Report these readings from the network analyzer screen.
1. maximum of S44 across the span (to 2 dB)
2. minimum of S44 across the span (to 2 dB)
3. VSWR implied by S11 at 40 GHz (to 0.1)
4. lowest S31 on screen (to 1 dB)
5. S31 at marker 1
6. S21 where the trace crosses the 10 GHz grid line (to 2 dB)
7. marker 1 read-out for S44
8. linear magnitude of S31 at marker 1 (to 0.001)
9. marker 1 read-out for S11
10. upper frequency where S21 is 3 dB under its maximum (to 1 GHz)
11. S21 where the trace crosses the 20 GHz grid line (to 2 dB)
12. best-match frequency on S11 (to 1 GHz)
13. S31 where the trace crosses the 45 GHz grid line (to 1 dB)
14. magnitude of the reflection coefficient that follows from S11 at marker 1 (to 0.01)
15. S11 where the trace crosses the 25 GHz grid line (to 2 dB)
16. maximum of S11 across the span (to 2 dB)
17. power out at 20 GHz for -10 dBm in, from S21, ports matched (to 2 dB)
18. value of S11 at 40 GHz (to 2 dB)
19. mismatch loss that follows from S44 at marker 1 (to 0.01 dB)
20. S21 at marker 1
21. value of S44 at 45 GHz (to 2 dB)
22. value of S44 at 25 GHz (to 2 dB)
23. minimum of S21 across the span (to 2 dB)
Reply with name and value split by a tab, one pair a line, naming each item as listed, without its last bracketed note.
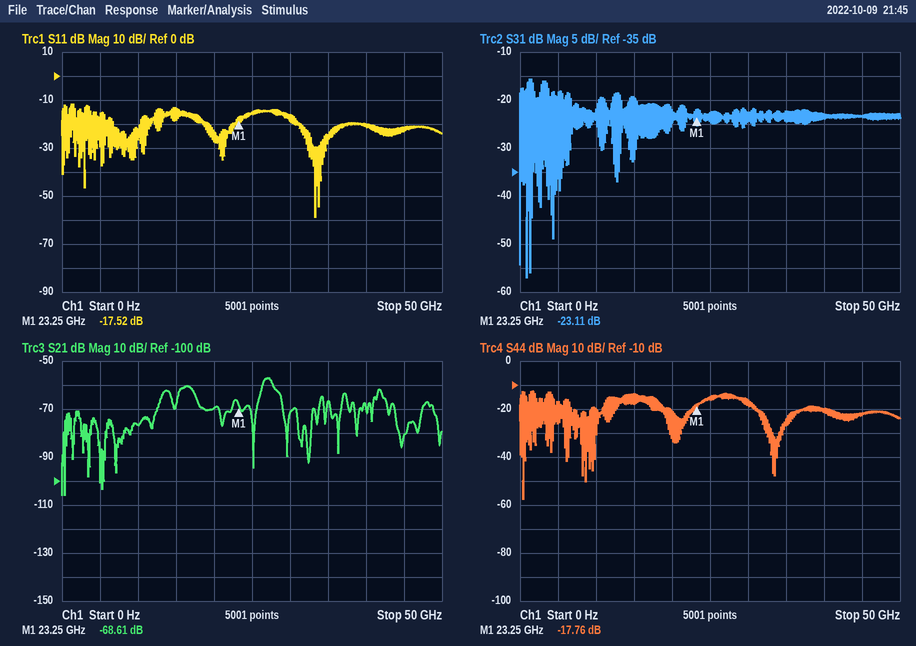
maximum of S44 across the span	-12 dB
minimum of S44 across the span	-58 dB
VSWR implied by S11 at 40 GHz	1.2
lowest S31 on screen	-57 dB
S31 at marker 1	-23.11 dB
S21 where the trace crosses the 10 GHz grid line	-76 dB
marker 1 read-out for S44	-17.76 dB
linear magnitude of S31 at marker 1	0.070
marker 1 read-out for S11	-17.52 dB
upper frequency where S21 is 3 dB under its maximum	28 GHz
S21 where the trace crosses the 20 GHz grid line	-70 dB
best-match frequency on S11	33 GHz
S31 where the trace crosses the 45 GHz grid line	-23 dB
magnitude of the reflection coefficient that follows from S11 at marker 1	0.13
S11 where the trace crosses the 25 GHz grid line	-16 dB
maximum of S11 across the span	-12 dB
power out at 20 GHz for -10 dBm in, from S21, ports matched	-80 dBm
value of S11 at 40 GHz	-20 dB
mismatch loss that follows from S44 at marker 1	0.07 dB
S21 at marker 1	-68.61 dB
value of S44 at 45 GHz	-22 dB
value of S44 at 25 GHz	-16 dB
minimum of S21 across the span	-106 dB
